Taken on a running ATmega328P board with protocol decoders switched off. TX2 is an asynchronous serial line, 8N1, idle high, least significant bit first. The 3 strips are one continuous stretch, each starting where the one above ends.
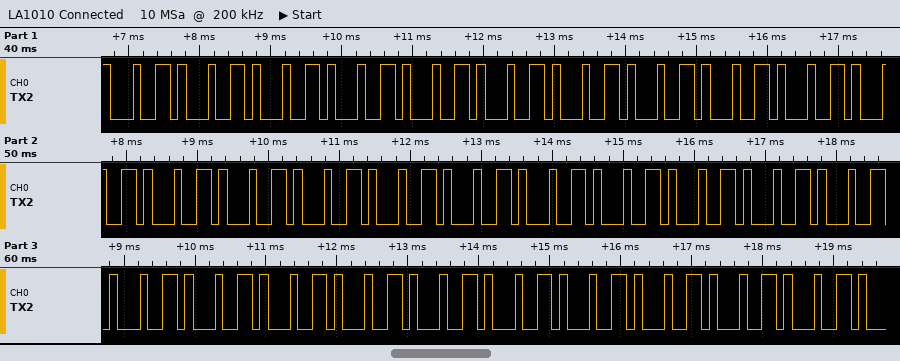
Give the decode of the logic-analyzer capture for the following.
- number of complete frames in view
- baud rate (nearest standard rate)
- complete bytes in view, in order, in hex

31
9600 baud
64 64 64 64 64 64 64 64 64 64 64 64 64 64 64 64 64 64 64 64 64 64 64 64 64 64 64 64 64 64 64
